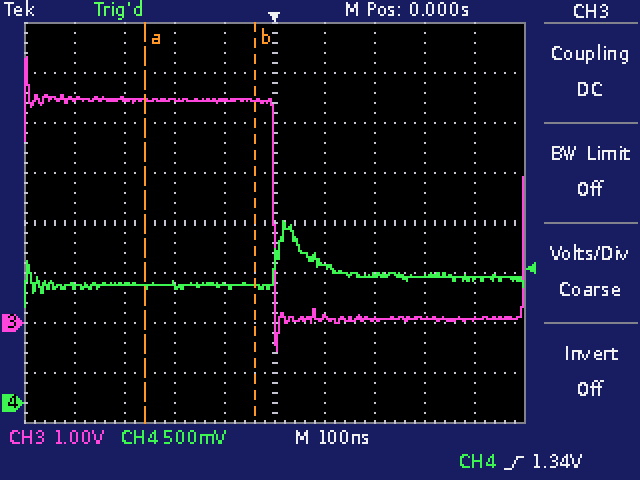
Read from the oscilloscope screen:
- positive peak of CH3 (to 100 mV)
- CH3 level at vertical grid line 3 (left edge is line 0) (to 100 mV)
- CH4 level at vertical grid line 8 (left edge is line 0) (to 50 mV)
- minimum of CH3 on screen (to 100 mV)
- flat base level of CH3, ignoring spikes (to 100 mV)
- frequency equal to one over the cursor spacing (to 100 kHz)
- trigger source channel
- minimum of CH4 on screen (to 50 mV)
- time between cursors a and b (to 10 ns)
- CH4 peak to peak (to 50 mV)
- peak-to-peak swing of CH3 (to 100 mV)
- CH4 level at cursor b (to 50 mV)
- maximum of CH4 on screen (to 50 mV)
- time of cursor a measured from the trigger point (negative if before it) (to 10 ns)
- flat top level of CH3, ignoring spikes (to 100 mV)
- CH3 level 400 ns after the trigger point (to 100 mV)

5.3 V
4.5 V
1.25 V
-600 mV
100 mV
4.5 MHz
CH4
950 mV
220 ns
850 mV
5.9 V
1.15 V
1.80 V
-260 ns
4.5 V
100 mV
